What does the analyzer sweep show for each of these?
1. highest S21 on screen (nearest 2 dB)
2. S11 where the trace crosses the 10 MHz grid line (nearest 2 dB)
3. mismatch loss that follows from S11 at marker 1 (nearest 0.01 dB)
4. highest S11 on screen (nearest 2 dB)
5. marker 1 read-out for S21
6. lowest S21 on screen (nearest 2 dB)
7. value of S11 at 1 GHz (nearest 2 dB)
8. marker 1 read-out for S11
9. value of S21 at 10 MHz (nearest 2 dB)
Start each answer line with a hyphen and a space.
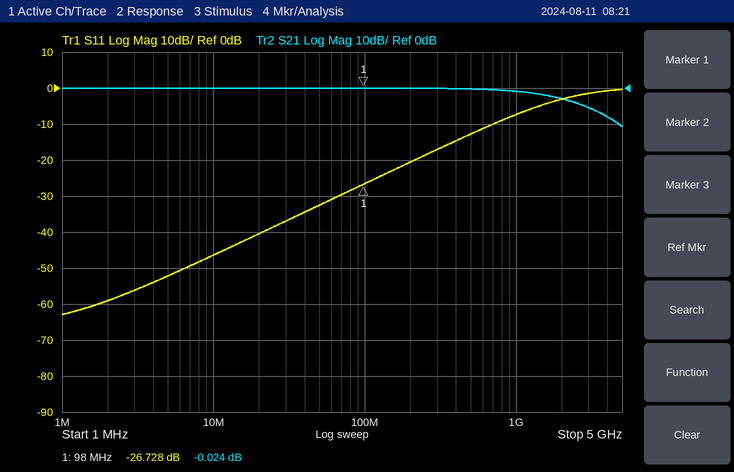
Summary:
- 0 dB
- -46 dB
- 0.01 dB
- 0 dB
- -0.024 dB
- -10 dB
- -8 dB
- -26.728 dB
- 0 dB
